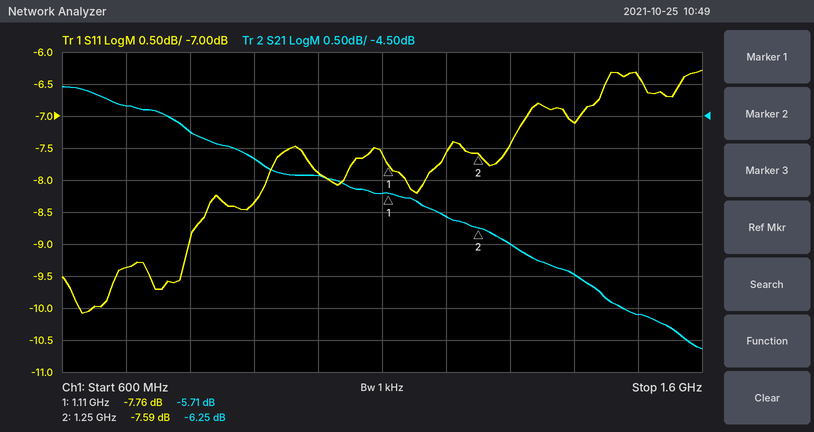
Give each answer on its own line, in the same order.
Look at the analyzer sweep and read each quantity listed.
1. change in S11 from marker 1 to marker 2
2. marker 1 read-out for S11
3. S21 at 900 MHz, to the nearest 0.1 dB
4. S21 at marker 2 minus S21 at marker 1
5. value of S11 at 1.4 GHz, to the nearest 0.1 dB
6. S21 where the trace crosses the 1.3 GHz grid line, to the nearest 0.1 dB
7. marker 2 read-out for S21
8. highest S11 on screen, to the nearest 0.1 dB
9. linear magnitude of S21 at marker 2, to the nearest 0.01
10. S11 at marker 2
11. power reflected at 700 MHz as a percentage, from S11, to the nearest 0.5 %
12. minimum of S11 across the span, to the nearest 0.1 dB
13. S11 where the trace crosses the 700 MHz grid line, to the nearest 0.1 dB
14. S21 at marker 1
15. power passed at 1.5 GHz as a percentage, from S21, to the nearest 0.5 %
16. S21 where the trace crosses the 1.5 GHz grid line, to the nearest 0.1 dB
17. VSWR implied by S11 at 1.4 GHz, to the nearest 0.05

0.17 dB
-7.76 dB
-5.2 dB
-0.54 dB
-7.1 dB
-6.5 dB
-6.25 dB
-6.3 dB
0.49
-7.59 dB
11.5 %
-10.1 dB
-9.4 dB
-5.71 dB
17.5 %
-7.6 dB
2.60
